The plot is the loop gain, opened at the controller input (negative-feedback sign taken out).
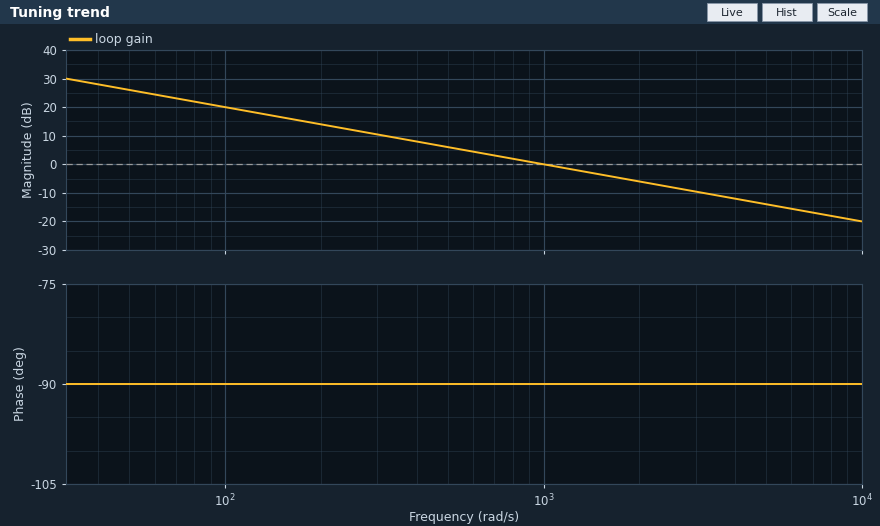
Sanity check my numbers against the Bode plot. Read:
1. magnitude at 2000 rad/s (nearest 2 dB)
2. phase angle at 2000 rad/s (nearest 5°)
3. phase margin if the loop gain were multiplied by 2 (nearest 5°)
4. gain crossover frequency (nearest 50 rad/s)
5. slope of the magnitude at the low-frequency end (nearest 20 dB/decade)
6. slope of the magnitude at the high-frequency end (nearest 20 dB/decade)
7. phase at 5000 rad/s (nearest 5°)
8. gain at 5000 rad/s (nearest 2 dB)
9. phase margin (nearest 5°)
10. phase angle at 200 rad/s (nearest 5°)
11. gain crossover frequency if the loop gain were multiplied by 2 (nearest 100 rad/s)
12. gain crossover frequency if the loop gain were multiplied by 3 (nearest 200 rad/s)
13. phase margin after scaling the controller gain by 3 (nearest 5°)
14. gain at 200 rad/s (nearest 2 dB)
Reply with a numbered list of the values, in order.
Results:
1. -6 dB
2. -90°
3. 90°
4. 1000 rad/s
5. -20 dB/decade
6. -20 dB/decade
7. -90°
8. -14 dB
9. 90°
10. -90°
11. 2000 rad/s
12. 3000 rad/s
13. 90°
14. 14 dB
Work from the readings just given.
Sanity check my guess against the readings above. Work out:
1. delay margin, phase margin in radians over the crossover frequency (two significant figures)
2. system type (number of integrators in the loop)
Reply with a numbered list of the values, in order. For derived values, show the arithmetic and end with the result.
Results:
1. 90 × π / 180 / 1000 = 0.0016 s
2. 1
